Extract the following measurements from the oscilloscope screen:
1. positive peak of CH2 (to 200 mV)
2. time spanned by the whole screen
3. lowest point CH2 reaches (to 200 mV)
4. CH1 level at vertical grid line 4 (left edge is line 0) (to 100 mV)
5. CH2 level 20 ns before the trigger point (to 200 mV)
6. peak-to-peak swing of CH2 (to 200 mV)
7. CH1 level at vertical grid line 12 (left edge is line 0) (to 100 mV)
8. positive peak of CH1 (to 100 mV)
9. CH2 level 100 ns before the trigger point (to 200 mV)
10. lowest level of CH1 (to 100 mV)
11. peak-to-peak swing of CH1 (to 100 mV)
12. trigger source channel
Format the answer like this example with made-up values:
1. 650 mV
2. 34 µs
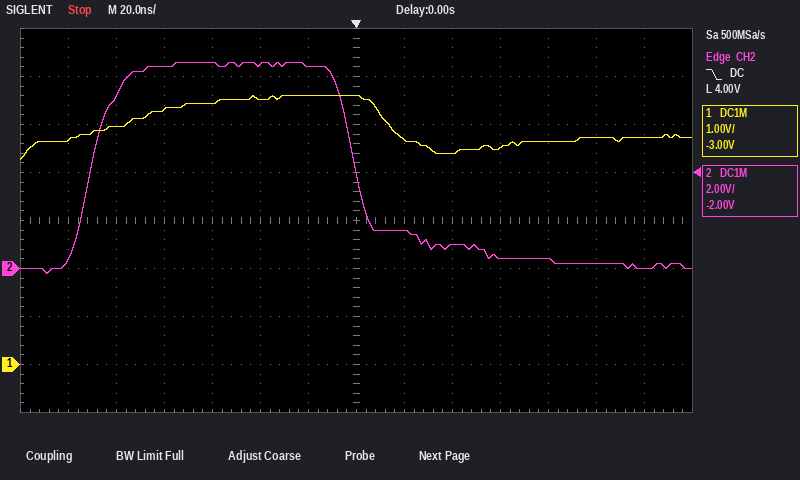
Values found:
1. 8.6 V
2. 280 ns
3. -200 mV
4. 5.4 V
5. 8.4 V
6. 8.8 V
7. 4.7 V
8. 5.6 V
9. 7.2 V
10. 4.3 V
11. 1.3 V
12. CH2
